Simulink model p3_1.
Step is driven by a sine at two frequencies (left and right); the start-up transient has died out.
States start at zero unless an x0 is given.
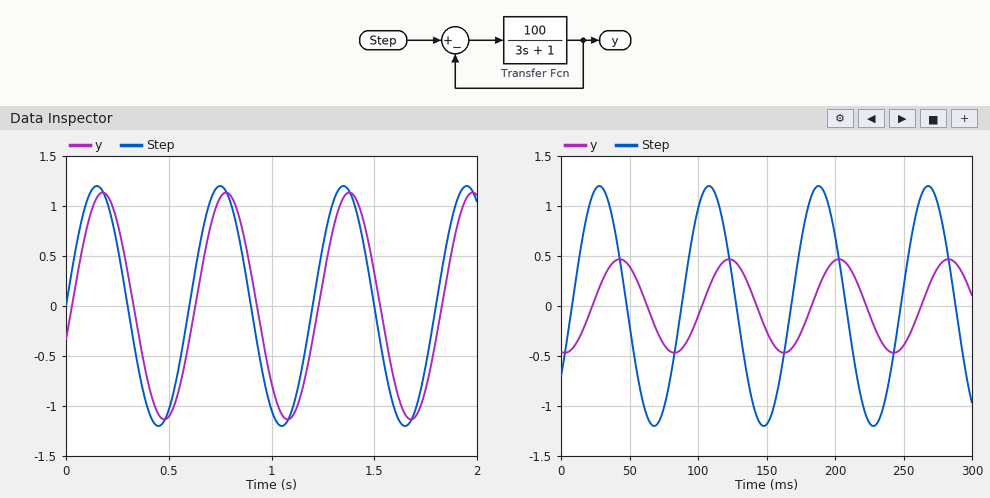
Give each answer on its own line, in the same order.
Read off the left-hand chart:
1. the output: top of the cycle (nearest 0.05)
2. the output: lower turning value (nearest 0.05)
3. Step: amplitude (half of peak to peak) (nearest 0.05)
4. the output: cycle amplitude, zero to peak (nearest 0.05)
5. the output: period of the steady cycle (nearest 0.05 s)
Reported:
1.15
-1.15
1.20
1.15
0.60 s
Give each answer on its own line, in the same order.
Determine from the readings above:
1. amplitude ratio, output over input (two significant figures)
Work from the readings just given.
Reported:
0.96
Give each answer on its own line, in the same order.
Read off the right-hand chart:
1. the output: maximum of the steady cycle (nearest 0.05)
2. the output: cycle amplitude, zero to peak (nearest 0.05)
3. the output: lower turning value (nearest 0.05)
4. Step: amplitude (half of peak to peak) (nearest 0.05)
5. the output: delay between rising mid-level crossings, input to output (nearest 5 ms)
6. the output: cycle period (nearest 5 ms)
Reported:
0.45
0.45
-0.45
1.20
15 ms
80 ms
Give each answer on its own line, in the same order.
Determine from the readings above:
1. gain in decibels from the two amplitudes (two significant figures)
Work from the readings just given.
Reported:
-8.5 dB
